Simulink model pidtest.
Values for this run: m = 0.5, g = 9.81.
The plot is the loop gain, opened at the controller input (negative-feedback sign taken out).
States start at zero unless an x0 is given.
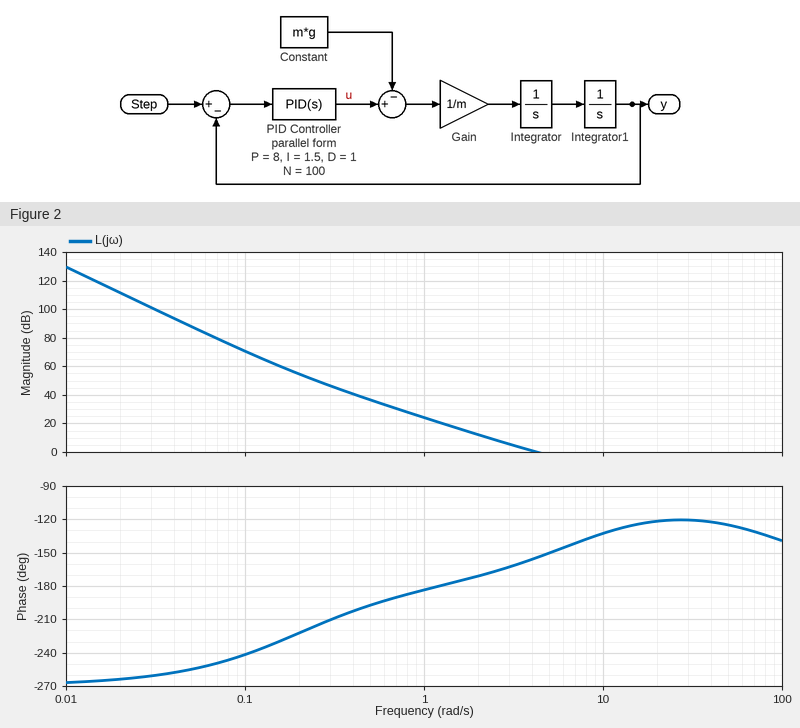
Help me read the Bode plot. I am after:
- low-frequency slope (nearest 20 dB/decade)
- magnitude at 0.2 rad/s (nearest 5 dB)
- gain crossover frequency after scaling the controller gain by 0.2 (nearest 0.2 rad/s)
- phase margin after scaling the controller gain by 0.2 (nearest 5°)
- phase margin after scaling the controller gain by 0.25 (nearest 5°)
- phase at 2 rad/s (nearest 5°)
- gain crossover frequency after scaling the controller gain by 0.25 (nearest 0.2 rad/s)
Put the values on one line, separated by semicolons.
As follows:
-60 dB/decade; 55 dB; 1.8 rad/s; 5°; 10°; -170°; 2.0 rad/s
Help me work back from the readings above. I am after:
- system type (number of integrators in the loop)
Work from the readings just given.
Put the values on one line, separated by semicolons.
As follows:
3
